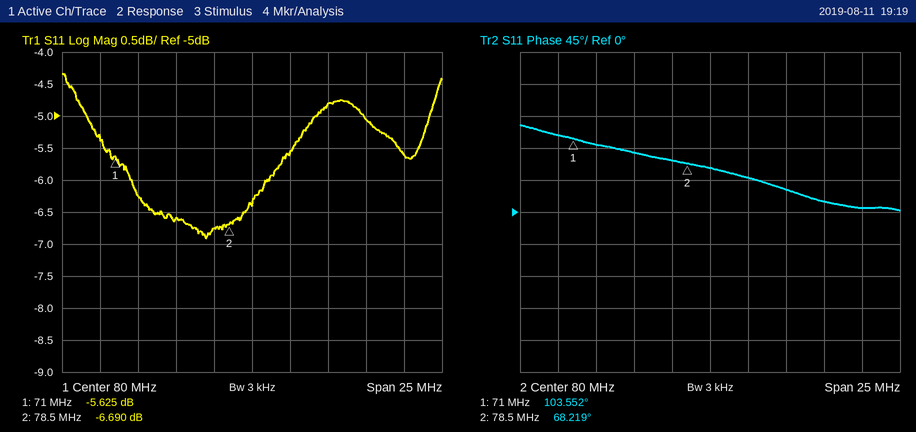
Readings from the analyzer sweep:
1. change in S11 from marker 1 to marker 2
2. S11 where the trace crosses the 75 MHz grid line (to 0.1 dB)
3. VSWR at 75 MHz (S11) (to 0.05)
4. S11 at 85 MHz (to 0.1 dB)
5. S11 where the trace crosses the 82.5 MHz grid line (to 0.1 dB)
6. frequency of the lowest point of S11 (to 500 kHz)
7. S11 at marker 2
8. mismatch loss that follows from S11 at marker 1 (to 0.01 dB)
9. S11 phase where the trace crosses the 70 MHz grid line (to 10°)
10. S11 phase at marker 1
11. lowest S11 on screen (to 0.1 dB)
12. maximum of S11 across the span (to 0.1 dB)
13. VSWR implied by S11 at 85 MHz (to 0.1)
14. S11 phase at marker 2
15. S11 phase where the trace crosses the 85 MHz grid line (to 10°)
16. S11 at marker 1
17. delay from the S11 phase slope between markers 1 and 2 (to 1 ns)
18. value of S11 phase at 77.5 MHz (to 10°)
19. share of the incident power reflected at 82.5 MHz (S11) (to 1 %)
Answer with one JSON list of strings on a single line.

["-1.065 dB", "-6.6 dB", "2.75", "-4.8 dB", "-5.6 dB", "77.0 MHz", "-6.690 dB", "1.39 dB", "110°", "103.552°", "-6.9 dB", "-4.3 dB", "3.7", "68.219°", "30°", "-5.625 dB", "13 ns", "70°", "28 %"]
